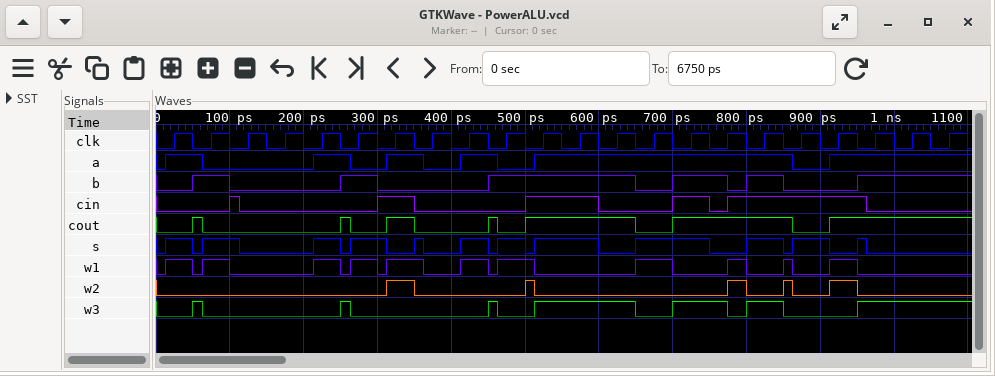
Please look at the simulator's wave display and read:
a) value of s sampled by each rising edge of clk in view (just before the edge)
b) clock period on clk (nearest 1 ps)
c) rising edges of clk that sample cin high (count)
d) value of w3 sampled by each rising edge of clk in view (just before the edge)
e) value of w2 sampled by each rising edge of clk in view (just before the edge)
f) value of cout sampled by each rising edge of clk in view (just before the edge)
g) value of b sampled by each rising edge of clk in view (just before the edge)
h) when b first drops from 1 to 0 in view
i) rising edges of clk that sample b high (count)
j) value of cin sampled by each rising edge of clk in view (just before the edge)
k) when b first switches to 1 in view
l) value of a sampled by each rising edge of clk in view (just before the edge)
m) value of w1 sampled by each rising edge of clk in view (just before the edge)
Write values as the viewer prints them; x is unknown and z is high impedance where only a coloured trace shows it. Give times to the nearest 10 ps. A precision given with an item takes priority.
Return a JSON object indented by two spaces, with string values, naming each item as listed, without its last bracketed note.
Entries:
{
  "value of s sampled by each rising edge of clk in view": "1 1 0 0 1 1 0 0 1 1 1 1 0 1 1 0 1 1 0 0 0 0",
  "clock period on clk": "50 ps",
  "rising edges of clk that sample cin high": "7",
  "value of w3 sampled by each rising edge of clk in view": "0 0 0 0 0 0 0 0 0 0 1 1 1 0 1 1 1 0 0 1 1 1",
  "value of w2 sampled by each rising edge of clk in view": "0 0 0 0 0 0 1 0 0 0 0 0 0 0 0 0 0 0 1 0 0 0",
  "value of cout sampled by each rising edge of clk in view": "0 0 0 0 0 0 1 0 0 0 1 1 1 0 1 1 1 0 1 1 1 1",
  "value of b sampled by each rising edge of clk in view": "0 1 0 0 0 1 0 0 0 1 1 1 1 0 1 1 1 0 0 1 1 1",
  "when b first drops from 1 to 0 in view": "100 ps",
  "rising edges of clk that sample b high": "12",
  "value of cin sampled by each rising edge of clk in view": "0 0 0 0 0 0 1 0 0 0 1 1 0 0 1 0 1 1 1 0 0 0",
  "when b first switches to 1 in view": "50 ps",
  "value of a sampled by each rising edge of clk in view": "1 0 0 0 1 0 1 0 1 0 1 1 1 1 1 1 1 0 1 1 1 1",
  "value of w1 sampled by each rising edge of clk in view": "1 1 0 0 1 1 1 0 1 1 0 0 0 1 0 0 0 0 1 0 0 0"
}
